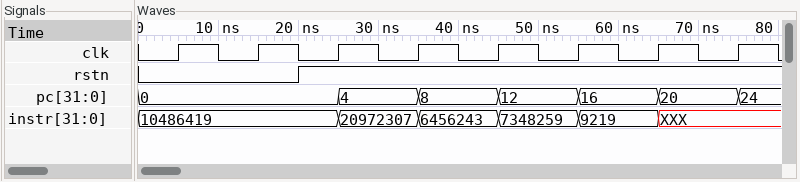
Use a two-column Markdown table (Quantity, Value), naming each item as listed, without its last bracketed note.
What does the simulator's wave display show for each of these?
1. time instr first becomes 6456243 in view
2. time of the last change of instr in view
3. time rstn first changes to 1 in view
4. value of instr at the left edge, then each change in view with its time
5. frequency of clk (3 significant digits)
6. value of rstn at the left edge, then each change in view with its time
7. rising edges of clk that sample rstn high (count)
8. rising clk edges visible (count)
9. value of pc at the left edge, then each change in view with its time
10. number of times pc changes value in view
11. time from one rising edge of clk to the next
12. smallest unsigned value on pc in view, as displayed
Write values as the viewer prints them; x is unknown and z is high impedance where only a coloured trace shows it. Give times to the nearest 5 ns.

| Quantity | Value |
|---|---|
| time instr first becomes 6456243 in view | 35 ns |
| time of the last change of instr in view | 65 ns |
| time rstn first changes to 1 in view | 20 ns |
| value of instr at the left edge, then each change in view with its time | 10486419, 20972307 at 25 ns, 6456243 at 35 ns, 7348259 at 45 ns, 9219 at 55 ns, XXX at 65 ns |
| frequency of clk | 100 MHz |
| value of rstn at the left edge, then each change in view with its time | 0, 1 at 20 ns |
| rising edges of clk that sample rstn high | 6 |
| rising clk edges visible | 8 |
| value of pc at the left edge, then each change in view with its time | 0, 4 at 25 ns, 8 at 35 ns, 12 at 45 ns, 16 at 55 ns, 20 at 65 ns, 24 at 75 ns |
| number of times pc changes value in view | 6 |
| time from one rising edge of clk to the next | 10 ns |
| smallest unsigned value on pc in view, as displayed | 0 |
